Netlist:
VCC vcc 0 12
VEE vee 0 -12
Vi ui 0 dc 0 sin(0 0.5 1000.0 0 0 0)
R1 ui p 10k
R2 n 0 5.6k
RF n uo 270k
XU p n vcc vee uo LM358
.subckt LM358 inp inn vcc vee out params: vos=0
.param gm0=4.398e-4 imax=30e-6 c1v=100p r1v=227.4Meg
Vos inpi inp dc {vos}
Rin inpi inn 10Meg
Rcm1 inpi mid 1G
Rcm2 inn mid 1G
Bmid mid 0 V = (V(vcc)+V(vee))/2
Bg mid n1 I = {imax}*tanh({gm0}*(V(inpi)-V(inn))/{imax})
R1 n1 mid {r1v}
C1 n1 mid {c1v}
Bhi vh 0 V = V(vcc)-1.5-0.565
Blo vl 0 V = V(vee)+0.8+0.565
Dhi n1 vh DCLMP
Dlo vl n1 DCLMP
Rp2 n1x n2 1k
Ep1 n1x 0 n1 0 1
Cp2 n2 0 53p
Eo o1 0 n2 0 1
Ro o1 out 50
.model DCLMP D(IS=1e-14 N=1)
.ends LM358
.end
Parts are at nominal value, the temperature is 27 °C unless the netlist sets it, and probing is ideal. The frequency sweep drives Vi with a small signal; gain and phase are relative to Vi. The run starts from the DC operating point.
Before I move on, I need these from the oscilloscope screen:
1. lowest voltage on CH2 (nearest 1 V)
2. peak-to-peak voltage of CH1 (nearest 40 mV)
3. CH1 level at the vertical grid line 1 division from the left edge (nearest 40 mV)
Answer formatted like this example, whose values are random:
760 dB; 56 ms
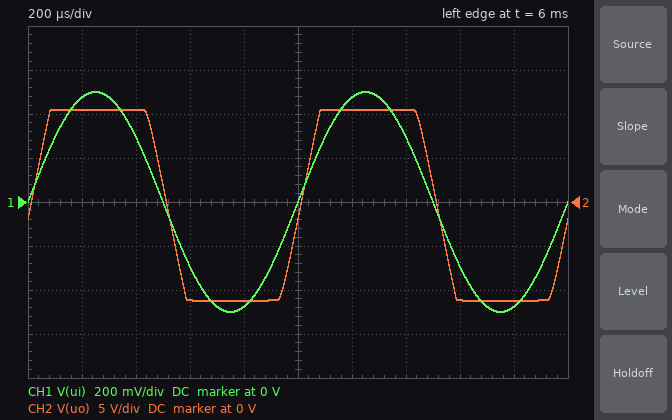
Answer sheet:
-11 V; 1.00 V; 480 mV
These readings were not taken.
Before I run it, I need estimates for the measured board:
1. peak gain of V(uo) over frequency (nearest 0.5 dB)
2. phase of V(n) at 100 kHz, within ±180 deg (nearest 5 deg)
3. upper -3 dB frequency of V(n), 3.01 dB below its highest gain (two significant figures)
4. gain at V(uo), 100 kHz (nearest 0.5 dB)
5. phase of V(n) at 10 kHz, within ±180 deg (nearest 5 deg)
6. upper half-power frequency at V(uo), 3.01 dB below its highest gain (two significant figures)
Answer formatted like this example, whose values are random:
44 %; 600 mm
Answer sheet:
34.0 dB; -85 deg; 14 kHz; 17.0 dB; -35 deg; 14 kHz
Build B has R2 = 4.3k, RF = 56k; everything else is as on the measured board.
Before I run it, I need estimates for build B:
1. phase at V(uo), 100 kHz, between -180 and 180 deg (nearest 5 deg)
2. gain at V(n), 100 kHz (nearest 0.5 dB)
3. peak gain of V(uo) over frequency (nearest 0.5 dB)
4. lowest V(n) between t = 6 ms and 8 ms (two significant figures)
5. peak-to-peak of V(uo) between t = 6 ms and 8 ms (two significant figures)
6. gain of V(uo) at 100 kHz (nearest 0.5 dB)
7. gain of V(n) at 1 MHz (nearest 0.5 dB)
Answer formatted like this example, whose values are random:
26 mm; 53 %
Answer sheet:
-65 deg; -7.0 dB; 23.0 dB; -500 mV; 14 V; 16.0 dB; -26.5 dB
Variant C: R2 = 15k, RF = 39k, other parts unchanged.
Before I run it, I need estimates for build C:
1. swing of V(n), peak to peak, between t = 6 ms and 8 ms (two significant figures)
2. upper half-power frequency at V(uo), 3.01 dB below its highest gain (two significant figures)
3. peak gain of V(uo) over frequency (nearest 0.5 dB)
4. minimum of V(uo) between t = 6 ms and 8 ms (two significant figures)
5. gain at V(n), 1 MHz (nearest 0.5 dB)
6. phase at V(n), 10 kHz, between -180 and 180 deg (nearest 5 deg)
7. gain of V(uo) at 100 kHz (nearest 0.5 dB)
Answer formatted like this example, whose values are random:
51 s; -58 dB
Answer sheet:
1.0 V; 210 kHz; 11.0 dB; -1.8 V; -14.5 dB; -5 deg; 10.0 dB
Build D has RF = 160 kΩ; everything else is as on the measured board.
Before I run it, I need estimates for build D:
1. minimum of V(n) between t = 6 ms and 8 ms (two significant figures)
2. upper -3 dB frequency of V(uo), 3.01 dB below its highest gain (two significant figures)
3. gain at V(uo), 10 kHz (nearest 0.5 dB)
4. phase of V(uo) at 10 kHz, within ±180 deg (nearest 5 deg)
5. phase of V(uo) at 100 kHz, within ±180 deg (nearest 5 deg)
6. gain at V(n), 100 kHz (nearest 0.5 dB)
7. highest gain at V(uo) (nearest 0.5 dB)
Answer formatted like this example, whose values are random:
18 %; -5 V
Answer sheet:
-380 mV; 24 kHz; 28.5 dB; -25 deg; -80 deg; -12.5 dB; 29.5 dB
